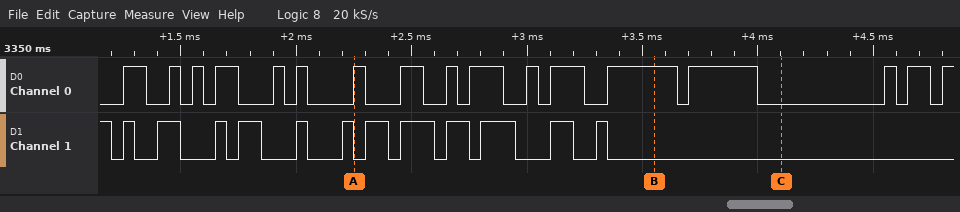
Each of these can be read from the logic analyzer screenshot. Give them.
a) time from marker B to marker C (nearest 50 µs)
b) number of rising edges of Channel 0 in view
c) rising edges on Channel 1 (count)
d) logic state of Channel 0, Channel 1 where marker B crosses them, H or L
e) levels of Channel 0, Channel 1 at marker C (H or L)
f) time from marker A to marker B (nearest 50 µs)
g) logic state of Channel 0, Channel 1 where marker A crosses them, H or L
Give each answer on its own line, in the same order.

550 µs
17
12
Channel 0=H, Channel 1=L
Channel 0=L, Channel 1=L
1300 µs
Channel 0=H, Channel 1=L
